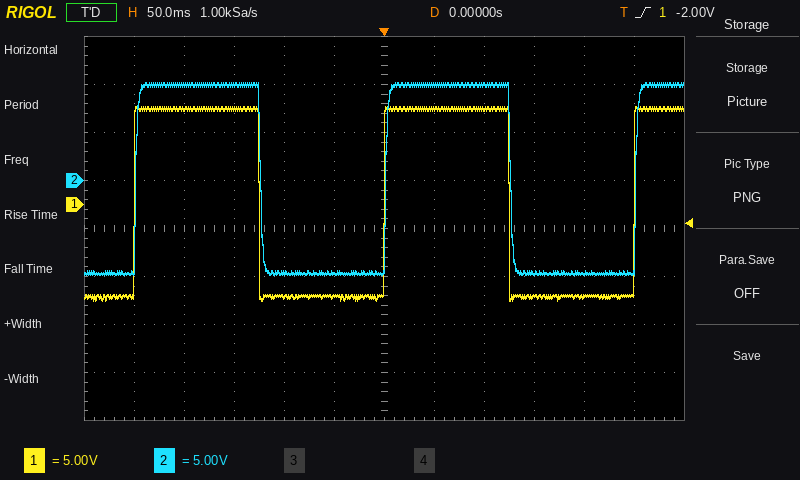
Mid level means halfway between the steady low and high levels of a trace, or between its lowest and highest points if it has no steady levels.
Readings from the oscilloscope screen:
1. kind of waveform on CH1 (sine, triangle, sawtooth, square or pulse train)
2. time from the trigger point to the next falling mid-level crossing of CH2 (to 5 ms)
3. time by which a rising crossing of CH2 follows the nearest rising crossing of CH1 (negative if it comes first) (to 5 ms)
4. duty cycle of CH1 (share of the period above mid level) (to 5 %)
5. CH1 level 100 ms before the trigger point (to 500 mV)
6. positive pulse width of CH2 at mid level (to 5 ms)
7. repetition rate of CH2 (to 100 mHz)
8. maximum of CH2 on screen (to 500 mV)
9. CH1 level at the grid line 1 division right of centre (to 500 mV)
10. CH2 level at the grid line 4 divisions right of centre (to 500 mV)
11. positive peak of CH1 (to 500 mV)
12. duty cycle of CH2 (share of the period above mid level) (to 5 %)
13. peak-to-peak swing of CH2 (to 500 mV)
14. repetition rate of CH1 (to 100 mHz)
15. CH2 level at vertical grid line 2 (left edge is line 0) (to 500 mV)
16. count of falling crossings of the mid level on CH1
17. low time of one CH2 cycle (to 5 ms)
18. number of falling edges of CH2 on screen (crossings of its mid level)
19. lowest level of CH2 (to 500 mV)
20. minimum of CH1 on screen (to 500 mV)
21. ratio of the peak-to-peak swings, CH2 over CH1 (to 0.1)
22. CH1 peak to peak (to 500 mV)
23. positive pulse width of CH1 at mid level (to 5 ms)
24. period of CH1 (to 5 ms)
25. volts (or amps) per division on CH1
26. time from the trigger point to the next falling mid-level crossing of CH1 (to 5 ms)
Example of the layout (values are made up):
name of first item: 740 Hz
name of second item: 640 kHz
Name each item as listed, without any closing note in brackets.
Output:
kind of waveform on CH1: square
time from the trigger point to the next falling mid-level crossing of CH2: 125 ms
time by which a rising crossing of CH2 follows the nearest rising crossing of CH1 (negative if it comes first): 0 ms
duty cycle of CH1 (share of the period above mid level): 50 %
CH1 level 100 ms before the trigger point: -9.5 V
positive pulse width of CH2 at mid level: 125 ms
repetition rate of CH2: 4.0 Hz
maximum of CH2 on screen: 10.0 V
CH1 level at the grid line 1 division right of centre: 10.0 V
CH2 level at the grid line 4 divisions right of centre: -9.5 V
positive peak of CH1: 10.0 V
duty cycle of CH2 (share of the period above mid level): 50 %
peak-to-peak swing of CH2: 20.0 V
repetition rate of CH1: 4.0 Hz
CH2 level at vertical grid line 2 (left edge is line 0): 10.0 V
count of falling crossings of the mid level on CH1: 2
low time of one CH2 cycle: 125 ms
number of falling edges of CH2 on screen: 2
lowest level of CH2: -10.0 V
minimum of CH1 on screen: -10.0 V
ratio of the peak-to-peak swings, CH2 over CH1: 1.0
CH1 peak to peak: 20.0 V
positive pulse width of CH1 at mid level: 125 ms
period of CH1: 250 ms
volts (or amps) per division on CH1: 5 V
time from the trigger point to the next falling mid-level crossing of CH1: 125 ms
